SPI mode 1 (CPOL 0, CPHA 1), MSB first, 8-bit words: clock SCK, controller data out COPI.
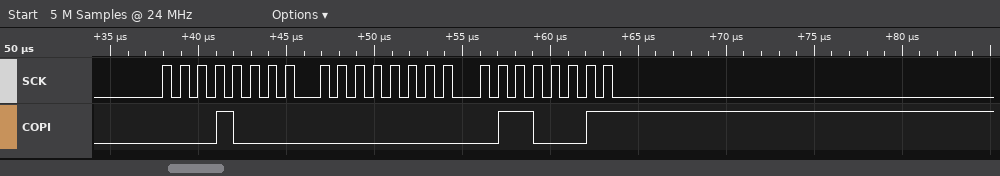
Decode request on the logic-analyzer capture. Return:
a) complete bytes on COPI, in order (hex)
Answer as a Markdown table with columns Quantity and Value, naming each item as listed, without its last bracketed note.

| Quantity | Value |
|---|---|
| complete bytes on COPI, in order | 0x10 0x00 0x63 |
